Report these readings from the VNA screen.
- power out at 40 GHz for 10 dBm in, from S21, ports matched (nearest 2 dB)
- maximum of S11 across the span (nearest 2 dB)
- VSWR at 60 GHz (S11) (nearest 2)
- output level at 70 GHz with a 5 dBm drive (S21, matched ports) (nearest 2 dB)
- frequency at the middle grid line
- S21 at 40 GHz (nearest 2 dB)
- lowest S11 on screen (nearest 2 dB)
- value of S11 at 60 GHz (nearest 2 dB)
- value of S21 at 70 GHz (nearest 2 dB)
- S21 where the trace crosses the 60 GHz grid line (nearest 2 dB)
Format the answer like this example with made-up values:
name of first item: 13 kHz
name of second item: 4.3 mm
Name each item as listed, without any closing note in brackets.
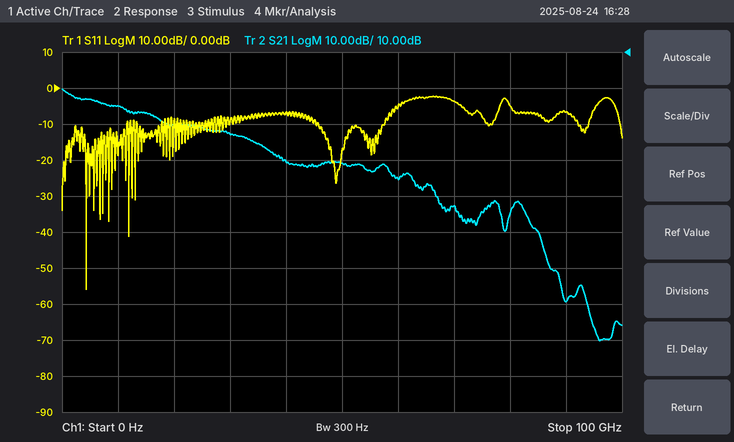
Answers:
power out at 40 GHz for 10 dBm in, from S21, ports matched: -10 dBm
maximum of S11 across the span: -2 dB
VSWR at 60 GHz (S11): 4
output level at 70 GHz with a 5 dBm drive (S21, matched ports): -28 dBm
frequency at the middle grid line: 50 GHz
S21 at 40 GHz: -20 dB
lowest S11 on screen: -56 dB
value of S11 at 60 GHz: -6 dB
value of S21 at 70 GHz: -32 dB
S21 where the trace crosses the 60 GHz grid line: -26 dB
